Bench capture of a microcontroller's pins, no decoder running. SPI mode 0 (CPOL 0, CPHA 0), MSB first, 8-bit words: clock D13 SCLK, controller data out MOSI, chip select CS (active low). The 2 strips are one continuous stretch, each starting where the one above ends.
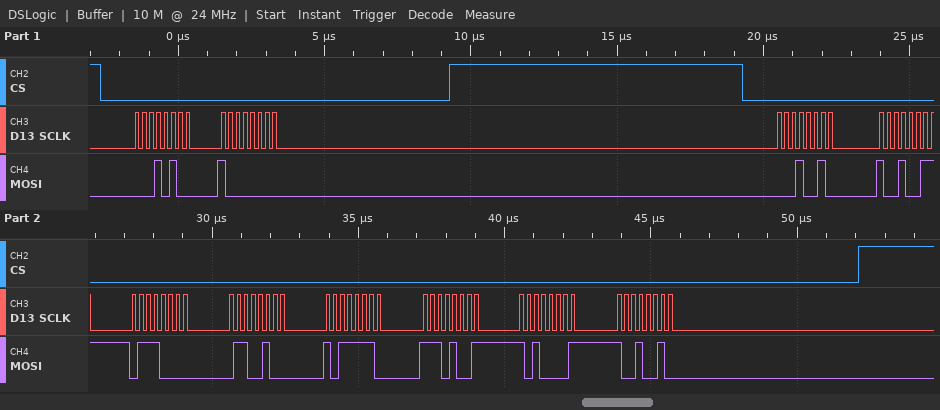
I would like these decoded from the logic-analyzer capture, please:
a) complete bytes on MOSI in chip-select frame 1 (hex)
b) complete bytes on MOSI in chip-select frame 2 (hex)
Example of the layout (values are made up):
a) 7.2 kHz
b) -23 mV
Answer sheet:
a) 14 80
b) 12 93 70 64 BE E9 A1 92
